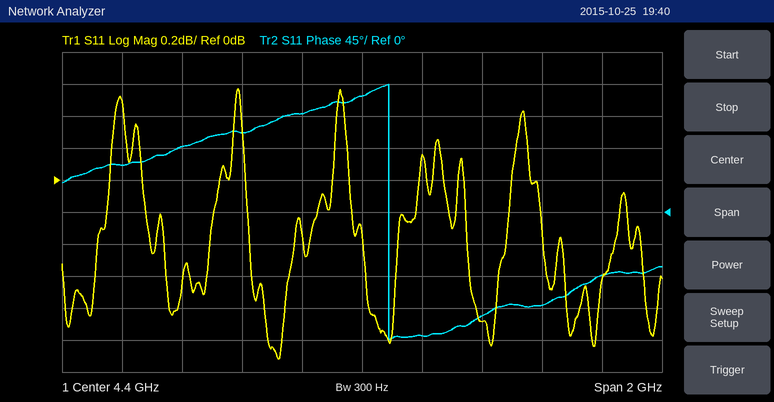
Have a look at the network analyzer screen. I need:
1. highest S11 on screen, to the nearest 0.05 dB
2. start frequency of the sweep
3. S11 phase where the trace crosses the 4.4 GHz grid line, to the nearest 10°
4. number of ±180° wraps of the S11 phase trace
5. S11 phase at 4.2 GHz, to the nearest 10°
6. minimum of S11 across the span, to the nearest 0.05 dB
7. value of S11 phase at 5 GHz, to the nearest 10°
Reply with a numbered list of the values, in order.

1. 0.55 dB
2. 3.4 GHz
3. 160°
4. 1
5. 140°
6. -1.10 dB
7. -130°
